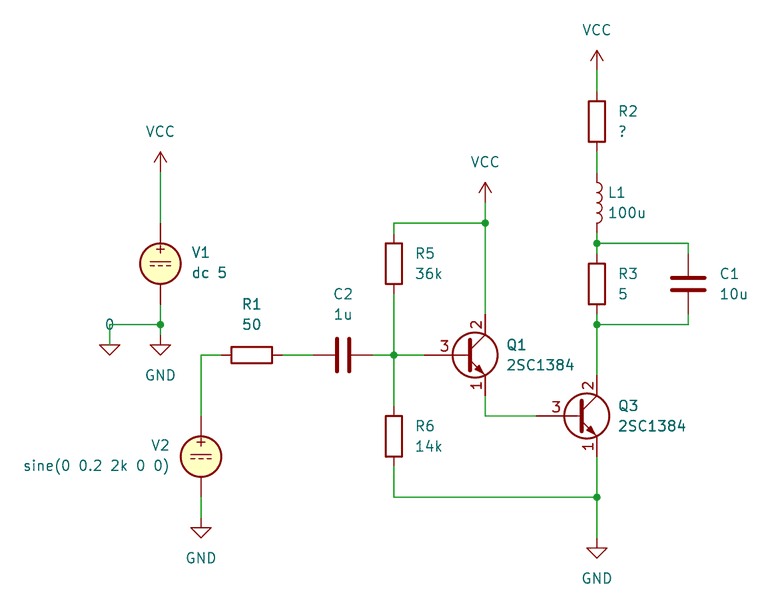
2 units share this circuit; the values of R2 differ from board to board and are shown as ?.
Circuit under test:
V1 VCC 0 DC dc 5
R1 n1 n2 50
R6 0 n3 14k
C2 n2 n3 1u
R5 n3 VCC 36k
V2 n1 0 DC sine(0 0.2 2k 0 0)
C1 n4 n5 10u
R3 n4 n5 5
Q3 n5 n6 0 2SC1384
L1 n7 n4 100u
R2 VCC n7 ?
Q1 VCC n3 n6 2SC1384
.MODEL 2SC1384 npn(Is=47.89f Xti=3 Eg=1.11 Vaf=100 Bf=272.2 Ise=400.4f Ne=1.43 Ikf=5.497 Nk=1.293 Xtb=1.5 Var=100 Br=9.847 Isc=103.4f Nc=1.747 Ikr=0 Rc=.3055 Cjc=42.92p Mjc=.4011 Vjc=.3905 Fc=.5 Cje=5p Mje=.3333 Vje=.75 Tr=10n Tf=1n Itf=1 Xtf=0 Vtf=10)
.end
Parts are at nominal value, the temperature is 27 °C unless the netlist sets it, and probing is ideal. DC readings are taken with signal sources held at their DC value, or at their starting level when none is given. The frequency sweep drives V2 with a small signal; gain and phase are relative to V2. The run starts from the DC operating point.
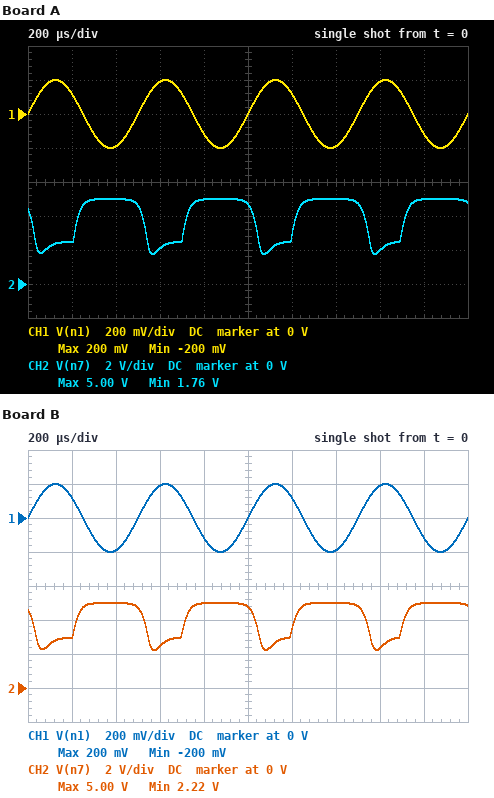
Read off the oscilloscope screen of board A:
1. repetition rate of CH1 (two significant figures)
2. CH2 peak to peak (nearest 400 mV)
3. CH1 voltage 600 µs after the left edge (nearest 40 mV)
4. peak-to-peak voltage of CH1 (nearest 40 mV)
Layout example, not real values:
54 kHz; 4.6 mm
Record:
2.0 kHz; 3.2 V; 200 mV; 400 mV
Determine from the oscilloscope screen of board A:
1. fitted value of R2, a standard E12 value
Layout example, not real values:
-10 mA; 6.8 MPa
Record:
5.6 Ω
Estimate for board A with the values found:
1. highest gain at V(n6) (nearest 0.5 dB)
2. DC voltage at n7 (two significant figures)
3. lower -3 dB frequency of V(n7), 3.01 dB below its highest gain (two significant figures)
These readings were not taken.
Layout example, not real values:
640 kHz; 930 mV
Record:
0.5 dB; 4.4 V; 240 kHz
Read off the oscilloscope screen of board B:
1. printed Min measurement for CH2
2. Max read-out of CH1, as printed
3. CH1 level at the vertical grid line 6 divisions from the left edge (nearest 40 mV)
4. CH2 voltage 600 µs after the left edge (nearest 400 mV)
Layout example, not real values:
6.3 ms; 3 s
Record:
2.22 V; 200 mV; 120 mV; 2.4 V
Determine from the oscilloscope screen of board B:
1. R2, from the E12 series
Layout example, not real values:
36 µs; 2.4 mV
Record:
3.9 Ω
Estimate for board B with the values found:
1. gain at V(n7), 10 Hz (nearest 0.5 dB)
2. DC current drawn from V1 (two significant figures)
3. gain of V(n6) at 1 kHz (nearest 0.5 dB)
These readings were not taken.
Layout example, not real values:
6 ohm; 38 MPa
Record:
8.0 dB; 110 mA; -5.5 dB
